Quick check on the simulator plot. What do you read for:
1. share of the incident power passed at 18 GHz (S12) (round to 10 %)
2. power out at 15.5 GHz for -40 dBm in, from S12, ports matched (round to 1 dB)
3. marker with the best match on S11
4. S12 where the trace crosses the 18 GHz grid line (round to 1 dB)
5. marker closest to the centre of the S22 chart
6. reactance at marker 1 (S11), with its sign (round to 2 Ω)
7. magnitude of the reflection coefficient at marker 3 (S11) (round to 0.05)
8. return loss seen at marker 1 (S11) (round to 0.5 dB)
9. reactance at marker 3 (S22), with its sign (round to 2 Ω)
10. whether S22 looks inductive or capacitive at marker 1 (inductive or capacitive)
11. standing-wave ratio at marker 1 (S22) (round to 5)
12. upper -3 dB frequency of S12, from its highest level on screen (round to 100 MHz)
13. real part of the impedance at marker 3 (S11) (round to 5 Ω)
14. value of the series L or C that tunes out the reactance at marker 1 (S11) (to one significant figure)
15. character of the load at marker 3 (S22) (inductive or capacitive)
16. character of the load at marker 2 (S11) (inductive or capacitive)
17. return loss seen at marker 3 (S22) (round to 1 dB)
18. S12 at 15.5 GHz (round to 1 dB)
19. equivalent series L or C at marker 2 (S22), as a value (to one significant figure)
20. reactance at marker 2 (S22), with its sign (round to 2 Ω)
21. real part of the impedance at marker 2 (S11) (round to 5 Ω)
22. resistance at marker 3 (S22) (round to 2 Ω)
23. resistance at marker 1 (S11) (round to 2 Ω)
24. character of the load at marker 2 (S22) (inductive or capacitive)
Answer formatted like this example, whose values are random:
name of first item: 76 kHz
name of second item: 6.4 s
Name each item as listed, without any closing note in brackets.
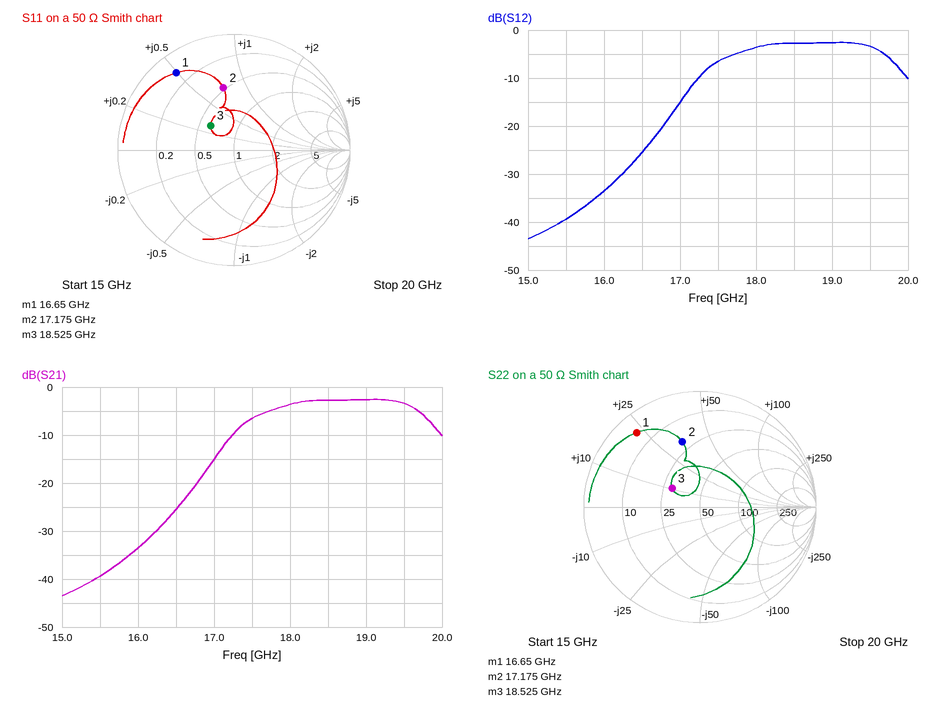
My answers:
share of the incident power passed at 18 GHz (S12): 40 %
power out at 15.5 GHz for -40 dBm in, from S12, ports matched: -79 dBm
marker with the best match on S11: marker 3
S12 where the trace crosses the 18 GHz grid line: -4 dB
marker closest to the centre of the S22 chart: marker 3
reactance at marker 1 (S11), with its sign: +24 Ω
magnitude of the reflection coefficient at marker 3 (S11): 0.30
return loss seen at marker 1 (S11): 1.5 dB
reactance at marker 3 (S22), with its sign: +10 Ω
whether S22 looks inductive or capacitive at marker 1: inductive
standing-wave ratio at marker 1 (S22): 10
upper -3 dB frequency of S12, from its highest level on screen: 19.7 GHz
real part of the impedance at marker 3 (S11): 30 Ω
value of the series L or C that tunes out the reactance at marker 1 (S11): 400 fF
character of the load at marker 3 (S22): inductive
character of the load at marker 2 (S11): inductive
return loss seen at marker 3 (S22): 11 dB
S12 at 15.5 GHz: -39 dB
equivalent series L or C at marker 2 (S22), as a value: 300 pH
reactance at marker 2 (S22), with its sign: +34 Ω
real part of the impedance at marker 2 (S11): 25 Ω
resistance at marker 3 (S22): 30 Ω
resistance at marker 1 (S11): 6 Ω
character of the load at marker 2 (S22): inductive
